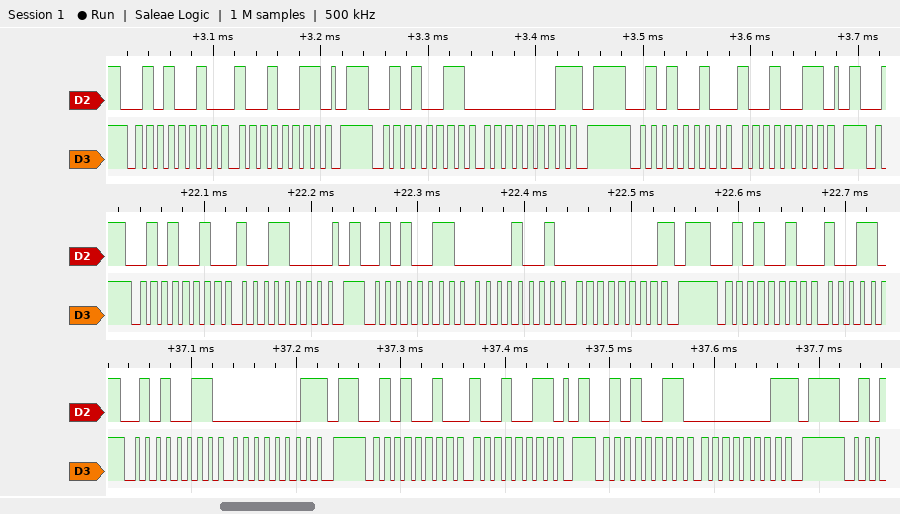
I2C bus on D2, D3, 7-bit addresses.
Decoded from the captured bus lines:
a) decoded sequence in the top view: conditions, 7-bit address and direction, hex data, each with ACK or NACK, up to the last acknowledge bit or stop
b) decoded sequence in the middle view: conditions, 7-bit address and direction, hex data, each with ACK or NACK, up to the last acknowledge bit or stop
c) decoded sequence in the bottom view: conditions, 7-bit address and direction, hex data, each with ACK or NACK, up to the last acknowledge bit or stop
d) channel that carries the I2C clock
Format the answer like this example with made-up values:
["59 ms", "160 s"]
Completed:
["start, address 29 write ACK, 93 ACK, stop, start, address 29 read ACK, 01 NACK, stop, start, address 29 write ACK, 93 ACK, stop", "start, address 29 write ACK, 98 ACK, stop, start, address 29 read ACK, 09 ACK, 00 NACK, stop, start, address 29 write ACK", "start, address 29 read ACK, 01 NACK, stop, start, address 29 write ACK, 93 ACK, stop, start, address 29 read ACK, 01 NACK, stop", "D3"]
